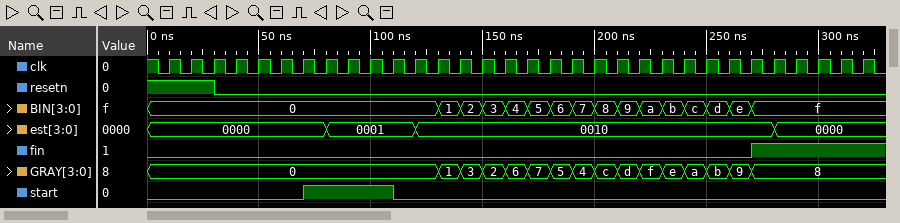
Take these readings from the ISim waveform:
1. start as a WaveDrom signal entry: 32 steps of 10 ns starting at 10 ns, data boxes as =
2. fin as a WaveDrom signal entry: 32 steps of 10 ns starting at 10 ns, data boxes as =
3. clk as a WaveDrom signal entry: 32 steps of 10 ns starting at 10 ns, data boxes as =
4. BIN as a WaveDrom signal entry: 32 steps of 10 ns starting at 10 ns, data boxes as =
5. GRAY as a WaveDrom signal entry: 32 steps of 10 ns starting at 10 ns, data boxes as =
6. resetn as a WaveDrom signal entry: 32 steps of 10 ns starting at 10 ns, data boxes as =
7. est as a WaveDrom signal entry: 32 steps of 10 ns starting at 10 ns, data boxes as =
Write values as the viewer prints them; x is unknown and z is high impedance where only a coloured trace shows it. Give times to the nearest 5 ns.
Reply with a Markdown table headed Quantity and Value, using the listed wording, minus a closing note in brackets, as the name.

| Quantity | Value |
|---|---|
| start as a WaveDrom signal entry: 32 steps of 10 ns starting at 10 ns, data boxes as = | {name: 'start', wave: '0.....1...0.....................'} |
| fin as a WaveDrom signal entry: 32 steps of 10 ns starting at 10 ns, data boxes as = | {name: 'fin', wave: '0.........................1.....'} |
| clk as a WaveDrom signal entry: 32 steps of 10 ns starting at 10 ns, data boxes as = | {name: 'clk', wave: 'p...............................'} |
| BIN as a WaveDrom signal entry: 32 steps of 10 ns starting at 10 ns, data boxes as = | {name: 'BIN', wave: '=...........===============.....', data: '0 1 2 3 4 5 6 7 8 9 a b c d e f'} |
| GRAY as a WaveDrom signal entry: 32 steps of 10 ns starting at 10 ns, data boxes as = | {name: 'GRAY', wave: '=...........===============.....', data: '0 1 3 2 6 7 5 4 c d f e a b 9 8'} |
| resetn as a WaveDrom signal entry: 32 steps of 10 ns starting at 10 ns, data boxes as = | {name: 'resetn', wave: '1.0.............................'} |
| est as a WaveDrom signal entry: 32 steps of 10 ns starting at 10 ns, data boxes as = | {name: 'est', wave: '=......=...=...............=....', data: '0000 0001 0010 0000'} |
